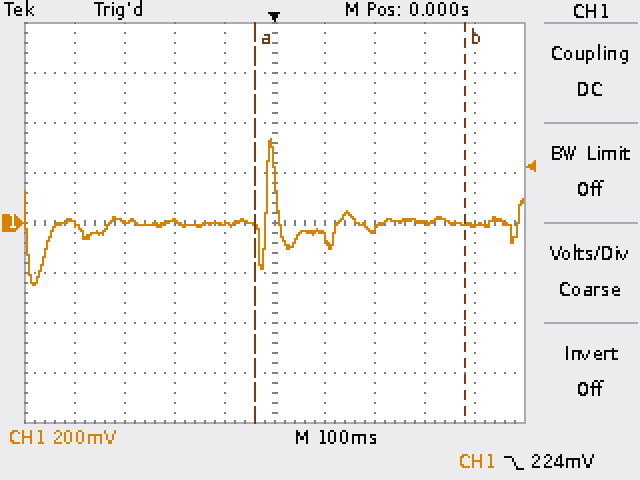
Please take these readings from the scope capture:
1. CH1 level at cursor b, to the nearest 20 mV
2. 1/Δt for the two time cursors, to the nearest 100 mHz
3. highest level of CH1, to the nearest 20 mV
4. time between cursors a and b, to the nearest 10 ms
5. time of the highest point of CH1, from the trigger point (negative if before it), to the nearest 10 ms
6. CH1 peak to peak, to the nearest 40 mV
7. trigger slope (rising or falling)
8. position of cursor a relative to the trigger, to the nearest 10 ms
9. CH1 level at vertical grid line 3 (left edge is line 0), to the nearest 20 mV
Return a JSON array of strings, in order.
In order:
["0 mV", "2.4 Hz", "340 mV", "420 ms", "-10 ms", "600 mV", "falling", "-40 ms", "0 mV"]
